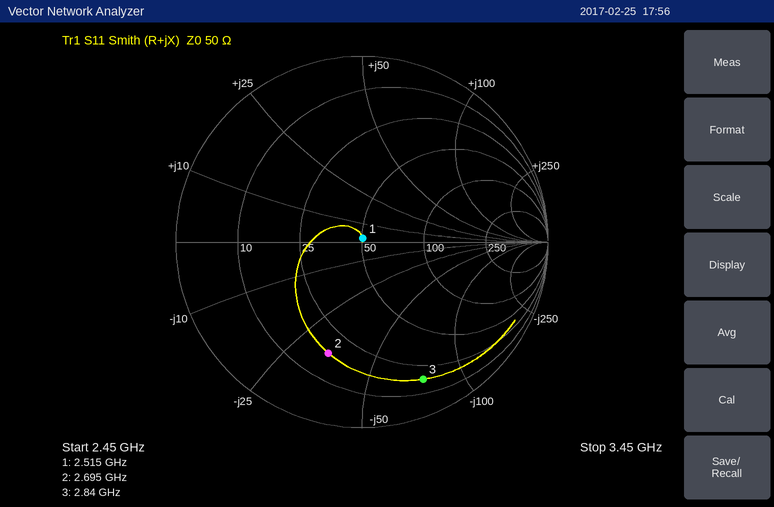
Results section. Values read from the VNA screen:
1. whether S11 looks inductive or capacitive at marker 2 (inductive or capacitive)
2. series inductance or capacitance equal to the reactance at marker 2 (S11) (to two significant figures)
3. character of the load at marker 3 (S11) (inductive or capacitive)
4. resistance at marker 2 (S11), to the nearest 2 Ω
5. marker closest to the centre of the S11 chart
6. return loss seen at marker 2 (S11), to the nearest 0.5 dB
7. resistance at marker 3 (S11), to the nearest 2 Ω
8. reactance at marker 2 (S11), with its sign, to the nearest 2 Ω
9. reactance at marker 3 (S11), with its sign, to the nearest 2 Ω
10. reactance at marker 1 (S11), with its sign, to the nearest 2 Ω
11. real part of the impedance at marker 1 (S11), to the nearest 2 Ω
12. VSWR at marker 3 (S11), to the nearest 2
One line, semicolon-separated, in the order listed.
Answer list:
capacitive; 1.7 pF; capacitive; 18 Ω; marker 1; 4.0 dB; 18 Ω; -34 Ω; -74 Ω; +2 Ω; 50 Ω; 10
